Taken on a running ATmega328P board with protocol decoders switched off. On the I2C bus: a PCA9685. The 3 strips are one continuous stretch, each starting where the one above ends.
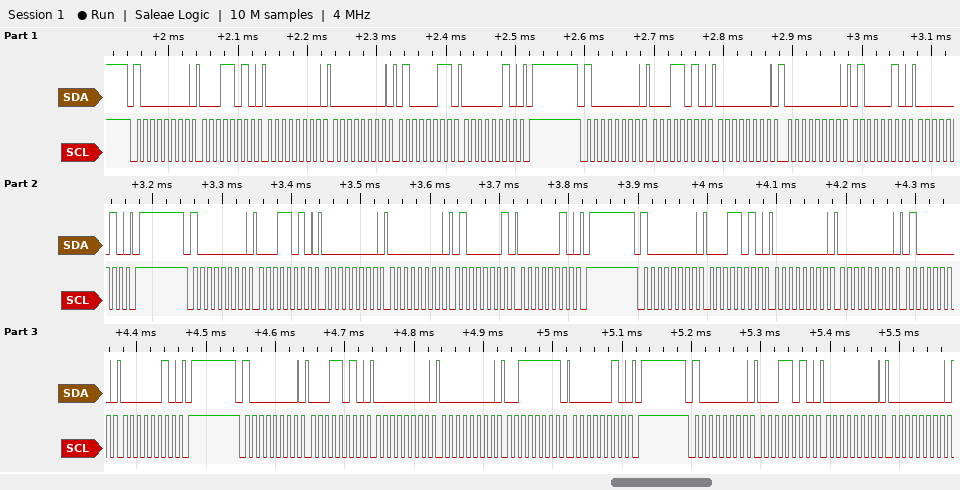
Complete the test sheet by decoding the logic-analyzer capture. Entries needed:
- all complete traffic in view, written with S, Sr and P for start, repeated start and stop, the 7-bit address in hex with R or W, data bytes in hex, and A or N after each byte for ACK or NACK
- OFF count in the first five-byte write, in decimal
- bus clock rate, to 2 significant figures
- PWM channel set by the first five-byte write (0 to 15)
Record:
S 40W A 1A A 00 A 00 A 43 A 02 A P S 40W A 1A A 00 A 00 A 42 A 02 A P S 40W A 1A A 00 A 00 A 41 A 02 A P S 40W A 1A A 00 A 00 A 40 A 02 A P S 40W A 1A A 00 A 00 A 3F A 02 A P S 40W A 1A A 00 A 00 A
579
100 kHz
5
